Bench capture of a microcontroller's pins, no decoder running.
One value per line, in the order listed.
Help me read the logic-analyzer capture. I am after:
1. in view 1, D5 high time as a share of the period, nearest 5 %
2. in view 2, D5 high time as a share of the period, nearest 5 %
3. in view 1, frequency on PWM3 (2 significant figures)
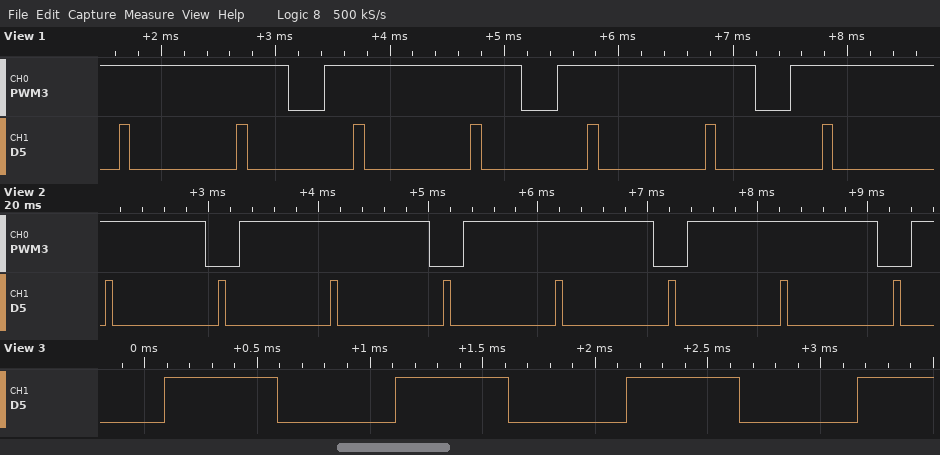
10 %
5 %
490 Hz
